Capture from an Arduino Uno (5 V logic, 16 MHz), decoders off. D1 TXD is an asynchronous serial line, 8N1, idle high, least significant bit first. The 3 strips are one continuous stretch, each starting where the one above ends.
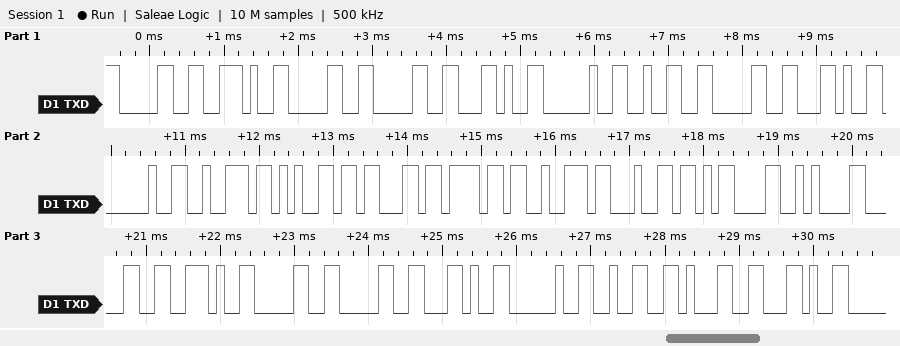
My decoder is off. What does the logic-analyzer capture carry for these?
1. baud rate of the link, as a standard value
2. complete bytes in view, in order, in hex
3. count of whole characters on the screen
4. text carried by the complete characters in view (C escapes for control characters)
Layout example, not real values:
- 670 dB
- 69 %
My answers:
- 9600 baud
- 30 2E 30 30 2C 20 32 30 2C 20 72 65 63 6F 72 64 0D 0A 30 2E 30 30 2C 20 32 31 2C
- 27
- "0.00, 20, record\r\n0.00, 21,"
